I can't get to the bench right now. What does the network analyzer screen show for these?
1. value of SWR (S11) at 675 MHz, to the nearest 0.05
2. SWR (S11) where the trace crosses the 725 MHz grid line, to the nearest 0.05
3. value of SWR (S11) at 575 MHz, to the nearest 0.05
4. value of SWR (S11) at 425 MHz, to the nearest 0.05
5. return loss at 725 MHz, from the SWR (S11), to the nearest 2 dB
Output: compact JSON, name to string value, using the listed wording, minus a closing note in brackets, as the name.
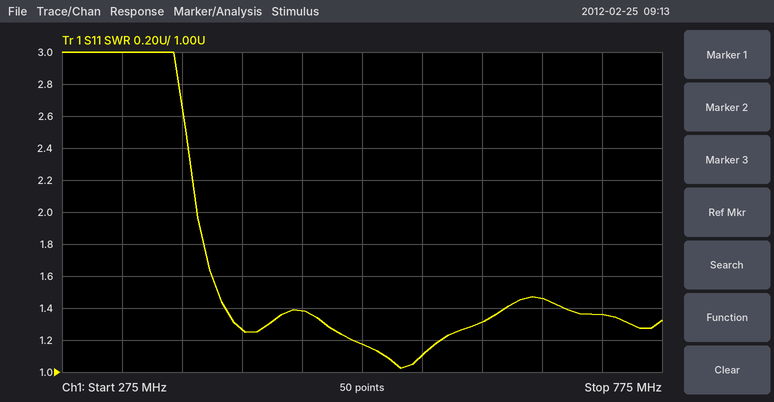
{"value of SWR (S11) at 675 MHz, to the nearest 0.05": "1.45", "SWR (S11) where the trace crosses the 725 MHz grid line, to the nearest 0.05": "1.35", "value of SWR (S11) at 575 MHz, to the nearest 0.05": "1.10", "value of SWR (S11) at 425 MHz, to the nearest 0.05": "1.25", "return loss at 725 MHz, from the SWR (S11), to the nearest 2 dB": "16 dB"}
